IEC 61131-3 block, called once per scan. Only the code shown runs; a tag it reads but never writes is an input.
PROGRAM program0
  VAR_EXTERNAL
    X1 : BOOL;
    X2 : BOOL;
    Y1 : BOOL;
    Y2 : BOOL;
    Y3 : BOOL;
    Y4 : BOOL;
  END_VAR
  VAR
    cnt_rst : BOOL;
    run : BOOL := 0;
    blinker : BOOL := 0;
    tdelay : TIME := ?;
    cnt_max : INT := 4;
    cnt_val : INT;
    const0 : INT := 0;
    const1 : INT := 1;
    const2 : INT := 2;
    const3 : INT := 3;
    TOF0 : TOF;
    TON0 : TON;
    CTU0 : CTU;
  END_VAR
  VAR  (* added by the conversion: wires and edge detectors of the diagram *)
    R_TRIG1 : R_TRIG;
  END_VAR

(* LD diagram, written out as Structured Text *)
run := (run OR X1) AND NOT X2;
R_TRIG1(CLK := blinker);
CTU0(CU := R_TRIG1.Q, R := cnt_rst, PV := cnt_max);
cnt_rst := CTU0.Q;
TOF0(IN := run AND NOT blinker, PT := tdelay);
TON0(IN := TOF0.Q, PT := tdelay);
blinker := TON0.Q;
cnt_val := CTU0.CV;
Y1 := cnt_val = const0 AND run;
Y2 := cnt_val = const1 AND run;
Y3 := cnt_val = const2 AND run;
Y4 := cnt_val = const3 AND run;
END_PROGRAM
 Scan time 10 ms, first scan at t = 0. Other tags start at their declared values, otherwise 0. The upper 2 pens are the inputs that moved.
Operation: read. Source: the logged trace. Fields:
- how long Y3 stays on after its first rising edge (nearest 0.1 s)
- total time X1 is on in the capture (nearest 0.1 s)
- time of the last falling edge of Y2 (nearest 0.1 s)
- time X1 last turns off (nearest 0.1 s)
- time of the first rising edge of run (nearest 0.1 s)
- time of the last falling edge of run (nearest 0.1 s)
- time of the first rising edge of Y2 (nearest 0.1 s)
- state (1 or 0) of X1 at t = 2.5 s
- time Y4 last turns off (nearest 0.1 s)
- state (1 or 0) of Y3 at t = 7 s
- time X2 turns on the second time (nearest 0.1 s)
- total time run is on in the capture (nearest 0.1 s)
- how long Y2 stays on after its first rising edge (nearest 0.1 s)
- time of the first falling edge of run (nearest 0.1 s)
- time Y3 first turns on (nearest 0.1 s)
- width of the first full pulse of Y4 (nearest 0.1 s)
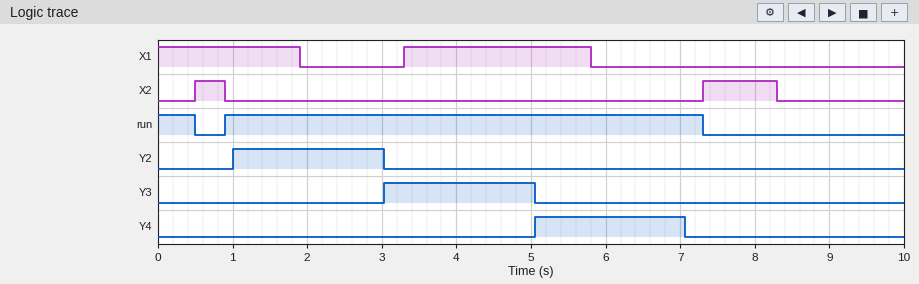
2.0 s
4.4 s
3.0 s
5.8 s
0.9 s
7.3 s
1.0 s
0
7.1 s
0
7.3 s
6.9 s
2.0 s
0.5 s
3.0 s
2.0 s
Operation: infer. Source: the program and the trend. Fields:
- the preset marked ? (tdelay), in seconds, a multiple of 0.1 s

1.0 s
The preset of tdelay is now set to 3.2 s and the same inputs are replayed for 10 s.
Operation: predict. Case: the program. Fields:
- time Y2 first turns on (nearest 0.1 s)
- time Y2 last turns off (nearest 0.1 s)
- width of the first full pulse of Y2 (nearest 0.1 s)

3.2 s
7.3 s
4.1 s
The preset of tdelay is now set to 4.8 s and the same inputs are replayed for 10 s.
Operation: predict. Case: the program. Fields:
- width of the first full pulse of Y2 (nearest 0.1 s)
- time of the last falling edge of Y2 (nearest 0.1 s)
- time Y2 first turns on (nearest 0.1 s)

2.5 s
7.3 s
4.8 s
